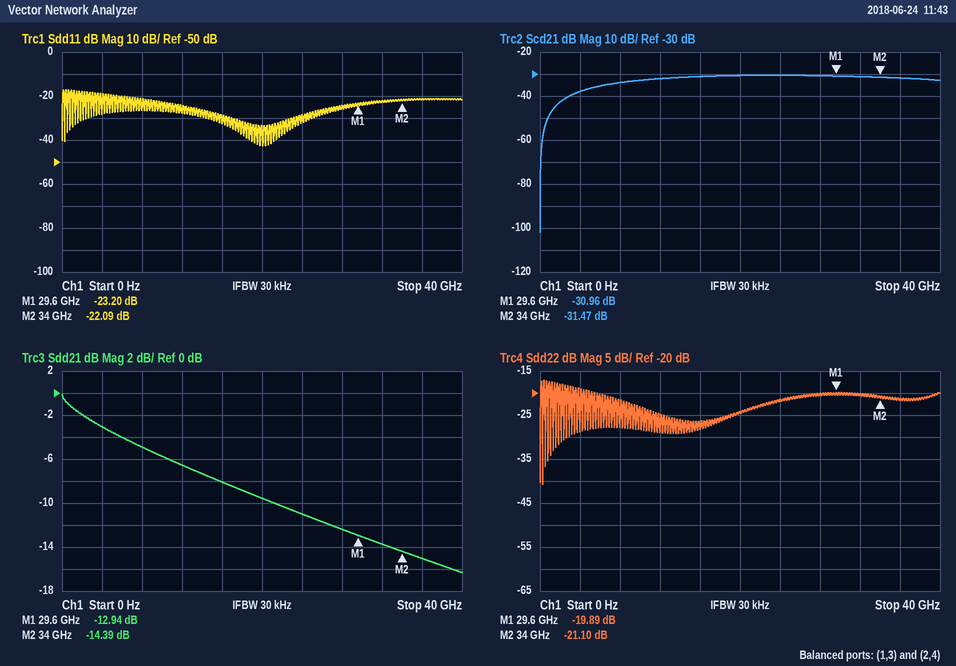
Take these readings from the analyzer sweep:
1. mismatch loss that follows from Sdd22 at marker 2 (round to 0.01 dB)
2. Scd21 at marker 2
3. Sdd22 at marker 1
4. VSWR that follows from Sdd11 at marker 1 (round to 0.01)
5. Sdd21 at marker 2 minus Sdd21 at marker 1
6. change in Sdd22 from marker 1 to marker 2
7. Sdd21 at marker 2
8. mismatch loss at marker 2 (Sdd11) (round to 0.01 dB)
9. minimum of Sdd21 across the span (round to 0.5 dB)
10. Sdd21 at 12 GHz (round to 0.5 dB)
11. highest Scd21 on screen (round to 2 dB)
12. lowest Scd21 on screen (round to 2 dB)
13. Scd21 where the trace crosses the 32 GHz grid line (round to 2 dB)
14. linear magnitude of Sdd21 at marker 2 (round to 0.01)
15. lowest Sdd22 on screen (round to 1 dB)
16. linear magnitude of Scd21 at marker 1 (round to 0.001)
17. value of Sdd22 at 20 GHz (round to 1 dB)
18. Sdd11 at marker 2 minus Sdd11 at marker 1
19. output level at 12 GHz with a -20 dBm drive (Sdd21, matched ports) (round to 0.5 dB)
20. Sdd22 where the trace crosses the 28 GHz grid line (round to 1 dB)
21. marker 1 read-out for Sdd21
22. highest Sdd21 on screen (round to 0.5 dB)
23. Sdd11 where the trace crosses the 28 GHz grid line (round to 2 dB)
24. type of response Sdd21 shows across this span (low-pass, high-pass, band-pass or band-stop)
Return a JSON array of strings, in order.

["0.03 dB", "-31.47 dB", "-19.89 dB", "1.15", "-1.45 dB", "-1.21 dB", "-14.39 dB", "0.03 dB", "-16.5 dB", "-6.5 dB", "-30 dB", "-102 dB", "-32 dB", "0.19", "-41 dB", "0.028", "-24 dB", "1.11 dB", "-26.5 dBm", "-20 dB", "-12.94 dB", "0.0 dB", "-24 dB", "low-pass"]
